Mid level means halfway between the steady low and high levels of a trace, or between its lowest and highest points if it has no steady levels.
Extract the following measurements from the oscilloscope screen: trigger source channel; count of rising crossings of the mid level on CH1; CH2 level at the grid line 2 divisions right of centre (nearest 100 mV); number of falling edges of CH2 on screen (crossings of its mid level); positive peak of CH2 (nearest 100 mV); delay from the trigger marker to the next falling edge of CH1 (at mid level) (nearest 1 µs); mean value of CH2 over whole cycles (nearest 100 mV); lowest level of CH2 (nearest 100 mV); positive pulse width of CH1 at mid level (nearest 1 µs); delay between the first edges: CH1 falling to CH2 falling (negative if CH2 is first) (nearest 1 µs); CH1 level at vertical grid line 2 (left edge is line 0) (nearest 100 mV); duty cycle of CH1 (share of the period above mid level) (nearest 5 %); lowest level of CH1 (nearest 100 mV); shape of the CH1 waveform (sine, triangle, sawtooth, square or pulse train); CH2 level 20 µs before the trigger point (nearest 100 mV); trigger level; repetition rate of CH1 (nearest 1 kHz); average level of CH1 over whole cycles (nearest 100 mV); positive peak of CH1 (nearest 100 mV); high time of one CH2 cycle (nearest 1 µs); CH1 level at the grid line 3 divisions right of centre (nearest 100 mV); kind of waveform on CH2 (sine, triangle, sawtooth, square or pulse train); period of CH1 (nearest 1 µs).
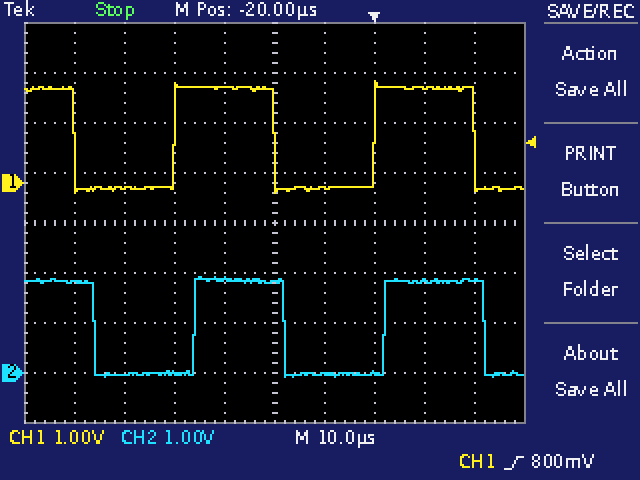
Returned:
CH1
2
0.0 V
3
1.9 V
20 µs
900 mV
-100 mV
20 µs
+4 µs
-100 mV
50 %
-200 mV
square
1.8 V
800 mV
25 kHz
900 mV
2.0 V
19 µs
1.9 V
square
40 µs
